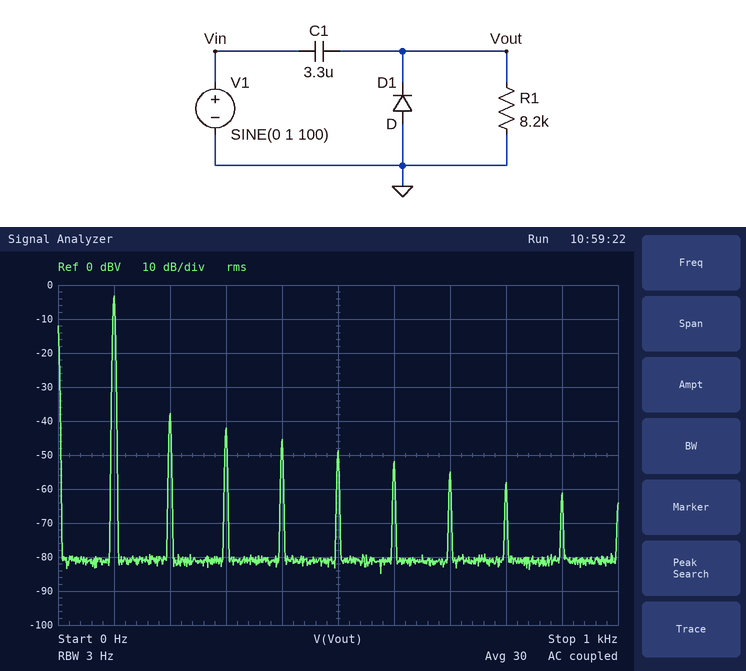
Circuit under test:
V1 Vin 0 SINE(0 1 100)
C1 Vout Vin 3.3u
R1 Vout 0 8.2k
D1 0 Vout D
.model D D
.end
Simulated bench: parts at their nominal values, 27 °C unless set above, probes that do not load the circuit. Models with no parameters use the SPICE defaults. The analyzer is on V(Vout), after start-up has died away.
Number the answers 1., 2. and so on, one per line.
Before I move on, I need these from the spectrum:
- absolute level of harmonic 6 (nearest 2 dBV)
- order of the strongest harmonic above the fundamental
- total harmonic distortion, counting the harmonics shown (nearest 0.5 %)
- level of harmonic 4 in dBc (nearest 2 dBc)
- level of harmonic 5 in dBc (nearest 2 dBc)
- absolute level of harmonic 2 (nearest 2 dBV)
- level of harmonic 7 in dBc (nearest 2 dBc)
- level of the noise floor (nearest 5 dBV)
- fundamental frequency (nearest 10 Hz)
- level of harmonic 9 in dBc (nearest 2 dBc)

1. -52 dBV
2. 2
3. 2.5 %
4. -42 dBc
5. -46 dBc
6. -38 dBV
7. -52 dBc
8. -80 dBV
9. 100 Hz
10. -58 dBc
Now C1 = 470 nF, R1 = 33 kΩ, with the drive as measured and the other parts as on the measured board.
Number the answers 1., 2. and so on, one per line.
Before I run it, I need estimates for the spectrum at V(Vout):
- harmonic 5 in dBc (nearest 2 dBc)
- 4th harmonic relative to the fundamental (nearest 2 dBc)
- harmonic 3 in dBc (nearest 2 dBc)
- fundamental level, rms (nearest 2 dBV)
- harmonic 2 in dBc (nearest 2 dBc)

1. -42 dBc
2. -38 dBc
3. -34 dBc
4. -4 dBV
5. -30 dBc
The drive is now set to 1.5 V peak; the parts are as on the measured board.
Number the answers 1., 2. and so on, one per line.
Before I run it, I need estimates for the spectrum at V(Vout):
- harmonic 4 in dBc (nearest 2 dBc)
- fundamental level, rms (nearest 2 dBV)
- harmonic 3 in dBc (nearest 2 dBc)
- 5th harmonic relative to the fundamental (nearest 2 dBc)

1. -38 dBc
2. 0 dBV
3. -36 dBc
4. -42 dBc
